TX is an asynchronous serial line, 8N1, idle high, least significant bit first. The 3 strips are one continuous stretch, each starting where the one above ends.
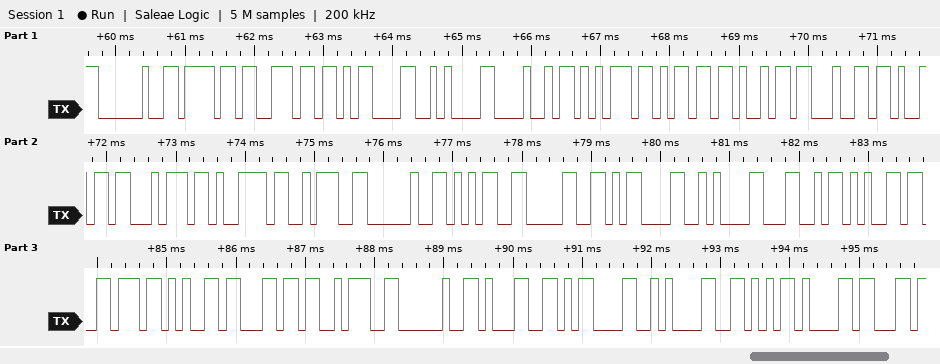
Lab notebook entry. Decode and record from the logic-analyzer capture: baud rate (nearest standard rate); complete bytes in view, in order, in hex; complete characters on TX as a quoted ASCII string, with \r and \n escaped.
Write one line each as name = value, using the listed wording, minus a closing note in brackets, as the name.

baud rate = 9600 baud
complete bytes in view, in order, in hex = 20 6F 6E 0D 0A 48 75 6D 69 64 69 74 79 3A 20 35 30 0D 0A 4C 65 76 65 6C 3A 20 31 0D 0A 56 61
complete characters on TX as a quoted ASCII string, with \r and \n escaped = " on\r\nHumidity: 50\r\nLevel: 1\r\nVa"
